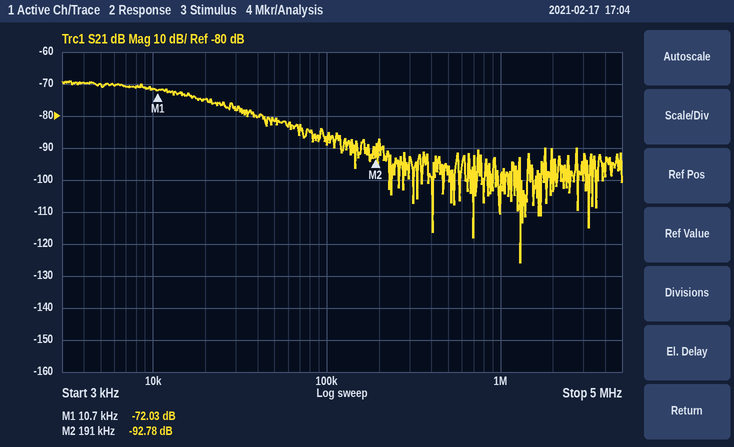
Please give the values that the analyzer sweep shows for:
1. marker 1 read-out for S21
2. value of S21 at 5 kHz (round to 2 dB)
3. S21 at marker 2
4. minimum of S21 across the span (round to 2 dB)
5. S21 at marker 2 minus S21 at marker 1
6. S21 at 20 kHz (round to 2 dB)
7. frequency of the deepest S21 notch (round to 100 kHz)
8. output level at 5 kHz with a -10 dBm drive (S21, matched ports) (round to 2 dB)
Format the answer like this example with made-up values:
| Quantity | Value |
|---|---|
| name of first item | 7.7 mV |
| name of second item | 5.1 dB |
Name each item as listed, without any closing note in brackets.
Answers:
| Quantity | Value |
|---|---|
| marker 1 read-out for S21 | -72.03 dB |
| value of S21 at 5 kHz | -70 dB |
| S21 at marker 2 | -92.78 dB |
| minimum of S21 across the span | -126 dB |
| S21 at marker 2 minus S21 at marker 1 | -20.75 dB |
| S21 at 20 kHz | -74 dB |
| frequency of the deepest S21 notch | 1.3 MHz |
| output level at 5 kHz with a -10 dBm drive (S21, matched ports) | -80 dBm |
